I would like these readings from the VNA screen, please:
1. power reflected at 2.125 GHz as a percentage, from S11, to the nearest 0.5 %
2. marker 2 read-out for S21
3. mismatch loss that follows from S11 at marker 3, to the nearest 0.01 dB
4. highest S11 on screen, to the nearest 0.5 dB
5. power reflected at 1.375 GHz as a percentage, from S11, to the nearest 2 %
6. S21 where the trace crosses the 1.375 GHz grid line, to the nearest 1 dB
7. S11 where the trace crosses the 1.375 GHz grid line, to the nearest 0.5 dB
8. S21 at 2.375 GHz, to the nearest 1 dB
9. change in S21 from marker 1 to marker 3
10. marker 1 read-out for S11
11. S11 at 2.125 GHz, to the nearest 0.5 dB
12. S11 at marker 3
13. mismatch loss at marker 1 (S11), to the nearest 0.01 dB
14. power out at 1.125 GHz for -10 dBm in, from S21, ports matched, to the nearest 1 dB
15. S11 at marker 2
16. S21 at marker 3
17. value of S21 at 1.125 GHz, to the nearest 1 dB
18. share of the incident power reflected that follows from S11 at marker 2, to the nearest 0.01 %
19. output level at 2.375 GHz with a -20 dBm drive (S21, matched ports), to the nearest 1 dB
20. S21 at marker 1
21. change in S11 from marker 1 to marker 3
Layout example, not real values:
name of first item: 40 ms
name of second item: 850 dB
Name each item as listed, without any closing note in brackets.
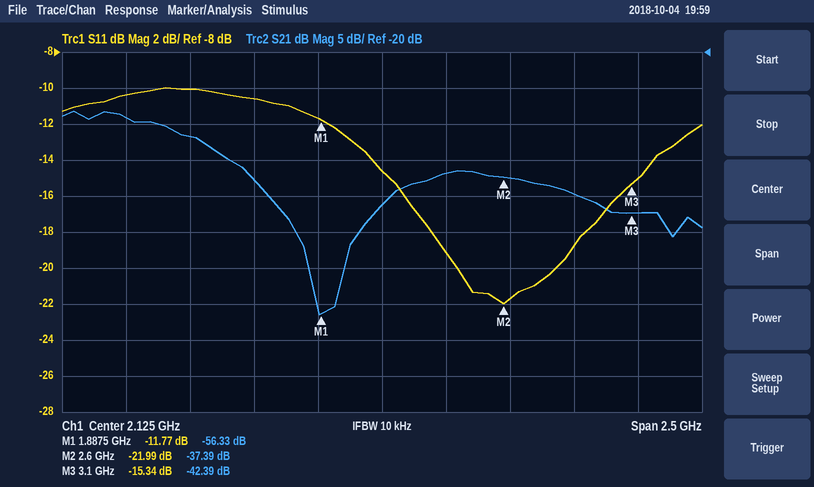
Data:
power reflected at 2.125 GHz as a percentage, from S11, to the nearest 0.5 %: 3.5 %
marker 2 read-out for S21: -37.39 dB
mismatch loss that follows from S11 at marker 3, to the nearest 0.01 dB: 0.13 dB
highest S11 on screen, to the nearest 0.5 dB: -10.0 dB
power reflected at 1.375 GHz as a percentage, from S11, to the nearest 2 %: 10 %
S21 where the trace crosses the 1.375 GHz grid line, to the nearest 1 dB: -32 dB
S11 where the trace crosses the 1.375 GHz grid line, to the nearest 0.5 dB: -10.0 dB
S21 at 2.375 GHz, to the nearest 1 dB: -37 dB
change in S21 from marker 1 to marker 3: 13.94 dB
marker 1 read-out for S11: -11.77 dB
S11 at 2.125 GHz, to the nearest 0.5 dB: -14.5 dB
S11 at marker 3: -15.34 dB
mismatch loss at marker 1 (S11), to the nearest 0.01 dB: 0.30 dB
power out at 1.125 GHz for -10 dBm in, from S21, ports matched, to the nearest 1 dB: -39 dBm
S11 at marker 2: -21.99 dB
S21 at marker 3: -42.39 dB
value of S21 at 1.125 GHz, to the nearest 1 dB: -29 dB
share of the incident power reflected that follows from S11 at marker 2, to the nearest 0.01 %: 0.63 %
output level at 2.375 GHz with a -20 dBm drive (S21, matched ports), to the nearest 1 dB: -57 dBm
S21 at marker 1: -56.33 dB
change in S11 from marker 1 to marker 3: -3.57 dB
